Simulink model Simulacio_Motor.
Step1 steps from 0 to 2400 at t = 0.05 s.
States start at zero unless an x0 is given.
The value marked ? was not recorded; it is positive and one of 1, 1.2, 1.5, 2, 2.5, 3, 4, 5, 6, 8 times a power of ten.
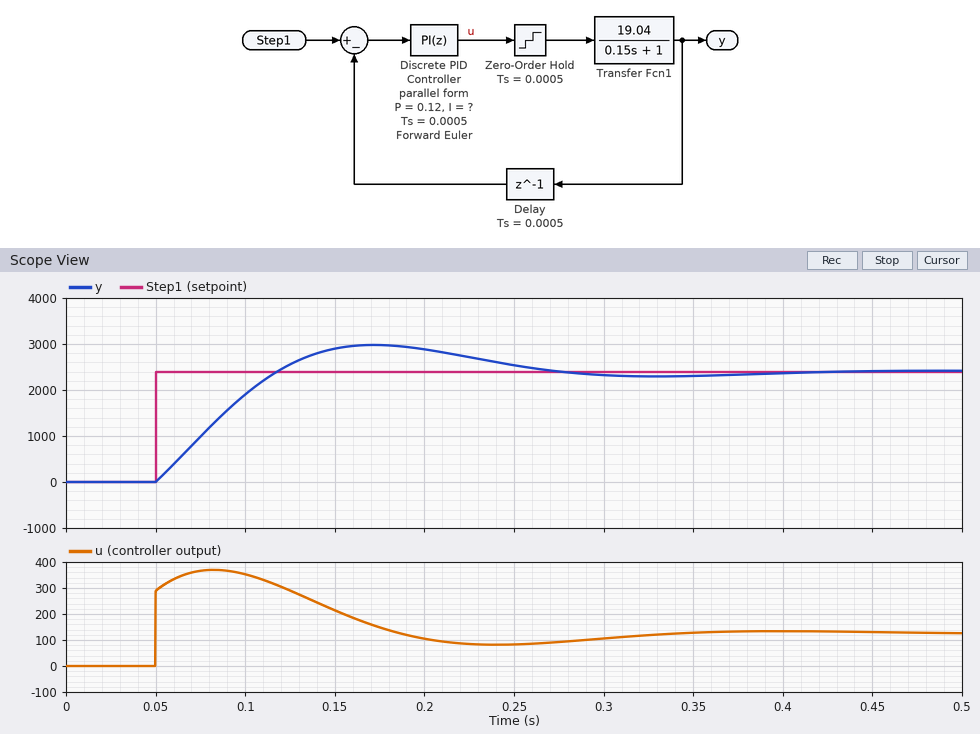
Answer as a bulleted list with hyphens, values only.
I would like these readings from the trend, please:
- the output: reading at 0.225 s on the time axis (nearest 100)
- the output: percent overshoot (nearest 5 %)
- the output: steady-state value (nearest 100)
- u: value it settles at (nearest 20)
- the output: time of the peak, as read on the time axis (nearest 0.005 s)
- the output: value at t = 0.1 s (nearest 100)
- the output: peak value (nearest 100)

- 2700
- 25 %
- 2400
- 120
- 0.170 s
- 1900
- 3000
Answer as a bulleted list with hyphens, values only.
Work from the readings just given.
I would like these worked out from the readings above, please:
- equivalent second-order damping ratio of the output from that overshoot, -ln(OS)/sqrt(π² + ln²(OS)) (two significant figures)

- 0.40
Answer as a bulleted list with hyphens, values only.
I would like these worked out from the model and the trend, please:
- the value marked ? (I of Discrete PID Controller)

- 4
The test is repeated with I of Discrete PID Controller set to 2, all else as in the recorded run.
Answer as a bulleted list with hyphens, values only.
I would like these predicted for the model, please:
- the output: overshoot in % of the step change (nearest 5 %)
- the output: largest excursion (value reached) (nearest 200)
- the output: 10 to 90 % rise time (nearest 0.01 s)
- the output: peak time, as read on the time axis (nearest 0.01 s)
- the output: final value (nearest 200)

- 10 %
- 2600
- 0.08 s
- 0.22 s
- 2400
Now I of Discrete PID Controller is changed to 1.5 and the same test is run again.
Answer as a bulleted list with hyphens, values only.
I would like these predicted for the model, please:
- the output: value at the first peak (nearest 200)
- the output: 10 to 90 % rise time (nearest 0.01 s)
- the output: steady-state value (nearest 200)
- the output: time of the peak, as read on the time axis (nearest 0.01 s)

- 2600
- 0.09 s
- 2400
- 0.26 s
